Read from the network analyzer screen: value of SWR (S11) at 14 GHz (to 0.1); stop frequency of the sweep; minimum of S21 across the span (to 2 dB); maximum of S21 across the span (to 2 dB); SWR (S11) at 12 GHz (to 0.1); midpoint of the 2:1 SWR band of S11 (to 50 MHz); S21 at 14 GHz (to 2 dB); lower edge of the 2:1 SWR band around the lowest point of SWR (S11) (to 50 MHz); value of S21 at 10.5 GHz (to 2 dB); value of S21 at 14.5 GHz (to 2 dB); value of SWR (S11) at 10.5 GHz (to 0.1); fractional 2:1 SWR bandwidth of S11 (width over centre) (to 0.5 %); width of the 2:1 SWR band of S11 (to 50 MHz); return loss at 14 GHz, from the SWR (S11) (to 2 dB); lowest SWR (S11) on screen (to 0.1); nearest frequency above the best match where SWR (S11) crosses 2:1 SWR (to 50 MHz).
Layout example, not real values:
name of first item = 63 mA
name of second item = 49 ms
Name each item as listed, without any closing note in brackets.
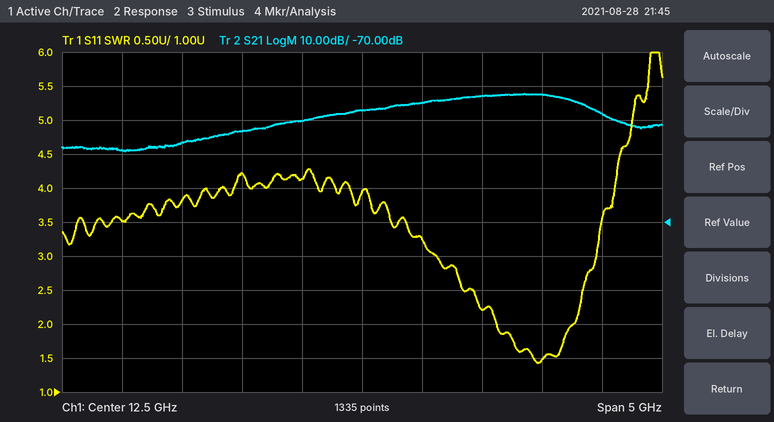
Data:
value of SWR (S11) at 14 GHz = 1.5
stop frequency of the sweep = 15 GHz
minimum of S21 across the span = -50 dB
maximum of S21 across the span = -32 dB
SWR (S11) at 12 GHz = 4.1
midpoint of the 2:1 SWR band of S11 = 13.95 GHz
S21 at 14 GHz = -32 dB
lower edge of the 2:1 SWR band around the lowest point of SWR (S11) = 13.60 GHz
value of S21 at 10.5 GHz = -48 dB
value of S21 at 14.5 GHz = -38 dB
value of SWR (S11) at 10.5 GHz = 3.5
fractional 2:1 SWR bandwidth of S11 (width over centre) = 4.5 %
width of the 2:1 SWR band of S11 = 650 MHz
return loss at 14 GHz, from the SWR (S11) = 14 dB
lowest SWR (S11) on screen = 1.4
nearest frequency above the best match where SWR (S11) crosses 2:1 SWR = 14.25 GHz
